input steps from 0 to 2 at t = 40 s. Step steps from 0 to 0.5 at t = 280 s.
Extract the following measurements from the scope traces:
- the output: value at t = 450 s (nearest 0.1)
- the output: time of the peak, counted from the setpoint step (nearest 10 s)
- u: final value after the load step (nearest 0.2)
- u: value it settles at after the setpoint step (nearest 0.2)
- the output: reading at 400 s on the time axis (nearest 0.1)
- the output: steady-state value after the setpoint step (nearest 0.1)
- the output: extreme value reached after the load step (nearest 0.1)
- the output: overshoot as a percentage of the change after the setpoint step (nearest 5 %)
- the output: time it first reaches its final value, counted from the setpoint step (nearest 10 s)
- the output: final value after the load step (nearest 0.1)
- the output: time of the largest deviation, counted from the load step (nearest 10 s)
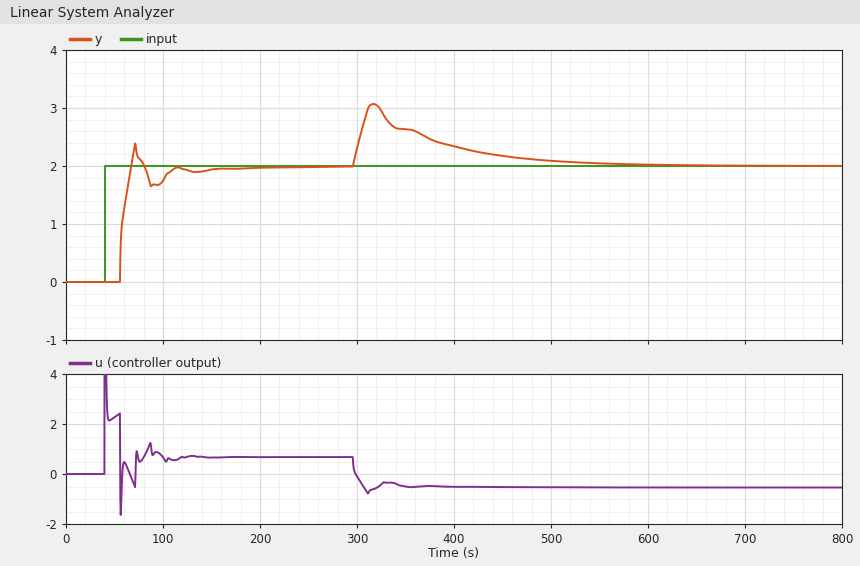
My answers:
2.2
30 s
-0.6
0.6
2.3
2.0
3.1
20 %
30 s
2.0
40 s
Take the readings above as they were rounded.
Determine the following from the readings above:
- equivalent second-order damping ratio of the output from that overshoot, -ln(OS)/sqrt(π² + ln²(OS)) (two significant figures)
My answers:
0.46
